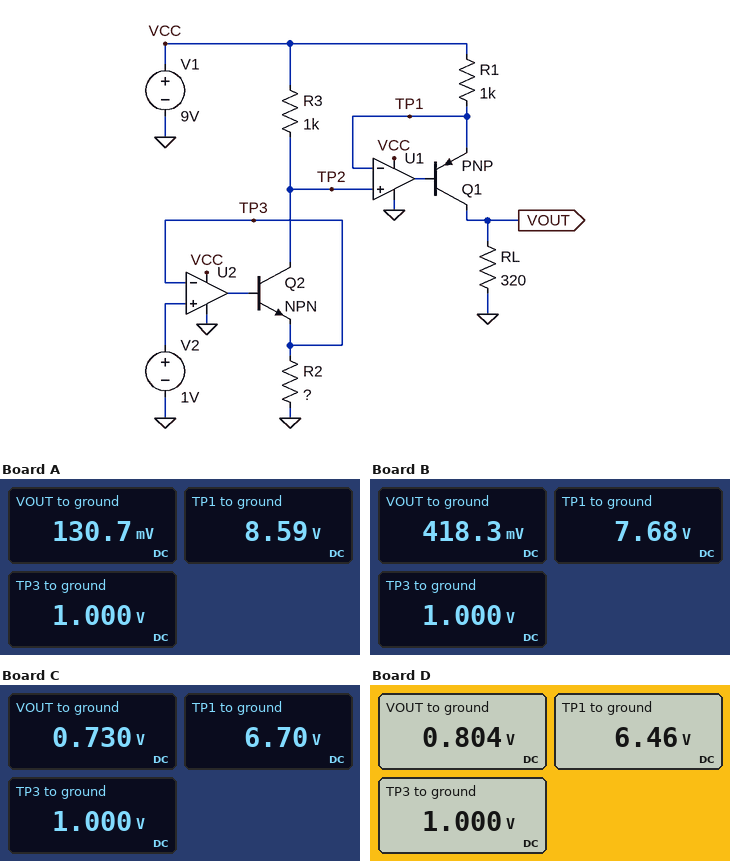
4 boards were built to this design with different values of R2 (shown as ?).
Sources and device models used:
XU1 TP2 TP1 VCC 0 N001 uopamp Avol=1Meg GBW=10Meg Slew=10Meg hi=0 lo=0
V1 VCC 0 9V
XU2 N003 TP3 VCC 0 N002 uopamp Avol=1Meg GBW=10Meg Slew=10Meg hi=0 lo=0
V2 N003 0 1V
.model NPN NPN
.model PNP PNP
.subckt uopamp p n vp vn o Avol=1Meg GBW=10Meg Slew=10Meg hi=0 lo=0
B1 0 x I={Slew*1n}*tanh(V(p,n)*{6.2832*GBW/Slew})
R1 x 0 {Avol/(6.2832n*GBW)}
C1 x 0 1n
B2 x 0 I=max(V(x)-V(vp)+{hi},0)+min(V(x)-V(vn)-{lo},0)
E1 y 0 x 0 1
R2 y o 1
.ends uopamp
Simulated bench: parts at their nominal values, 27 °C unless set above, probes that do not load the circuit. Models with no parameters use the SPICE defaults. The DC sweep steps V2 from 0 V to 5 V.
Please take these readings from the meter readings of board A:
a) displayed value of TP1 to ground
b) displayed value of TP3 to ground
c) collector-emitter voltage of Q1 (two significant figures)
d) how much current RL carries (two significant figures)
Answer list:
8.59 V
1.000 V
-8.5 V
410 µA
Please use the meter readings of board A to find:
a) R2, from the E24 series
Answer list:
2.4 kΩ
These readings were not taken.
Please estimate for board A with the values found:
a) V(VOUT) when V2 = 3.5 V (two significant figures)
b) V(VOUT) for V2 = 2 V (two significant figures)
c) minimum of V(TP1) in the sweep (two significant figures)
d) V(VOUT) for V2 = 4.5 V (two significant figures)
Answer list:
460 mV
260 mV
6.9 V
590 mV
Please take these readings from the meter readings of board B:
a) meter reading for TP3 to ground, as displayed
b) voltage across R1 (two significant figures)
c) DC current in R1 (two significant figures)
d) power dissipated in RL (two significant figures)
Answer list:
1.000 V
1.3 V
1.3 mA
550 µW
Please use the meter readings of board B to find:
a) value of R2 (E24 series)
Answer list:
750 Ω
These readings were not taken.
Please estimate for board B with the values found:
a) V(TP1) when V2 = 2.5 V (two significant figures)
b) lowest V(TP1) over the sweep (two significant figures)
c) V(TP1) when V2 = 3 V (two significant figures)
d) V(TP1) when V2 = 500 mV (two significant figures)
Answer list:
5.7 V
4.0 V
5.0 V
8.3 V
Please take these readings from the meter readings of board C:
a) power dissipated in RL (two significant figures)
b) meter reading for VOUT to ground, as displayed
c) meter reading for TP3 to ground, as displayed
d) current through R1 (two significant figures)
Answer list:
1.7 mW
0.730 V
1.000 V
2.3 mA
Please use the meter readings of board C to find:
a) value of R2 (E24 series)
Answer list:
430 Ω
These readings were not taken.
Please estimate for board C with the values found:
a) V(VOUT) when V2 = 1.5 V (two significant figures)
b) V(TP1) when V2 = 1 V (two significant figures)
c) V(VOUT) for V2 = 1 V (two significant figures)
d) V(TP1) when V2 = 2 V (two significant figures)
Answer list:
1.1 V
6.7 V
730 mV
4.4 V
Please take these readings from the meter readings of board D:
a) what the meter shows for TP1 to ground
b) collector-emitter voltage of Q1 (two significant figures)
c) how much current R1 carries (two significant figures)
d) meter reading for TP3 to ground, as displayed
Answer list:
6.46 V
-5.7 V
2.5 mA
1.000 V
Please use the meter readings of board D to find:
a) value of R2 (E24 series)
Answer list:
390 Ω
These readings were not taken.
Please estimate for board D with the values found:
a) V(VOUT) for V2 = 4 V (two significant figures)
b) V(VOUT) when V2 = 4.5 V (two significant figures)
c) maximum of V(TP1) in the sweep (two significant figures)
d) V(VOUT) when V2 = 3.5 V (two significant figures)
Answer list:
1.6 V
1.4 V
9.0 V
1.7 V
